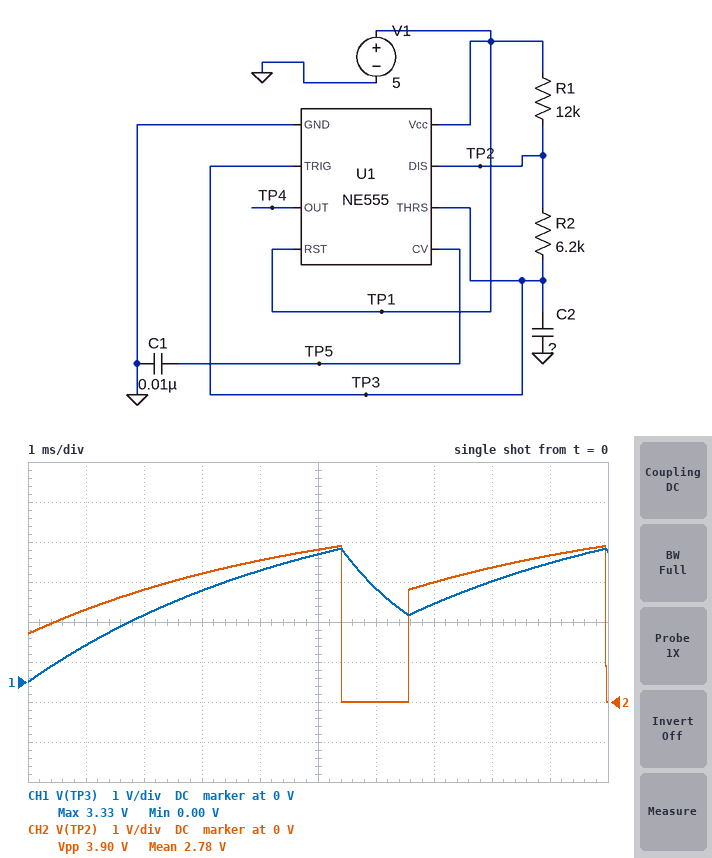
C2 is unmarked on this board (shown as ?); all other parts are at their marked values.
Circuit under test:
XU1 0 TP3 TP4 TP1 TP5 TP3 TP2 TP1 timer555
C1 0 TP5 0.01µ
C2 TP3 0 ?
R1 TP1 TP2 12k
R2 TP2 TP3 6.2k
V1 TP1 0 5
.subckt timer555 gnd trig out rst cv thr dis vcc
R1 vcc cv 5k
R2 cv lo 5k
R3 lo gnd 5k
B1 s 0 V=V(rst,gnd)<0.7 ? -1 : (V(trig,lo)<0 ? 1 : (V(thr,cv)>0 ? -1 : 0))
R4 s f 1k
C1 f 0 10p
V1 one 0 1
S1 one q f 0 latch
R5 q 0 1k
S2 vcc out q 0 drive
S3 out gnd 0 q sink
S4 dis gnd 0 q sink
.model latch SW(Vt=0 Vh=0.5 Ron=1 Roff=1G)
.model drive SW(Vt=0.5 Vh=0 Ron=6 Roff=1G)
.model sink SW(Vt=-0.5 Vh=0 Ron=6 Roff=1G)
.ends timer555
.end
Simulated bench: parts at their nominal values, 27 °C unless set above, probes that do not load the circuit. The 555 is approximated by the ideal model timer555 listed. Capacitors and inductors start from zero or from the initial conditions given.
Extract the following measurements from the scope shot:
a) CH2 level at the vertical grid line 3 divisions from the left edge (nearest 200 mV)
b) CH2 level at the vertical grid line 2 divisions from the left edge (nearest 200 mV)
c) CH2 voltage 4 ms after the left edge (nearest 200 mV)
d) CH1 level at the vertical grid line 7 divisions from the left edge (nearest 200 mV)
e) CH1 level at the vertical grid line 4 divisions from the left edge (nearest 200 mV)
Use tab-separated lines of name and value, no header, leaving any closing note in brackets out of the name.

CH2 level at the vertical grid line 3 divisions from the left edge	3.2 V
CH2 level at the vertical grid line 2 divisions from the left edge	2.8 V
CH2 voltage 4 ms after the left edge	3.6 V
CH1 level at the vertical grid line 7 divisions from the left edge	2.0 V
CH1 level at the vertical grid line 4 divisions from the left edge	2.8 V
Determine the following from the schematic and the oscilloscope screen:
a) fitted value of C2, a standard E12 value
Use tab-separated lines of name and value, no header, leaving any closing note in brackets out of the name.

fitted value of C2, a standard E12 value	270 nF
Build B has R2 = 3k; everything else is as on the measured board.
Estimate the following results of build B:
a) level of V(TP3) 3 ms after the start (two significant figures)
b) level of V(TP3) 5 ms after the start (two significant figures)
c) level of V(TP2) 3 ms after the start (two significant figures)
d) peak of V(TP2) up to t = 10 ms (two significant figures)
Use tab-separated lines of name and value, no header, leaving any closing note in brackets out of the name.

level of V(TP3) 3 ms after the start	2.6 V
level of V(TP3) 5 ms after the start	1.7 V
level of V(TP2) 3 ms after the start	3.1 V
peak of V(TP2) up to t = 10 ms	3.7 V
